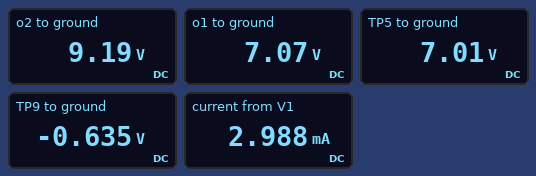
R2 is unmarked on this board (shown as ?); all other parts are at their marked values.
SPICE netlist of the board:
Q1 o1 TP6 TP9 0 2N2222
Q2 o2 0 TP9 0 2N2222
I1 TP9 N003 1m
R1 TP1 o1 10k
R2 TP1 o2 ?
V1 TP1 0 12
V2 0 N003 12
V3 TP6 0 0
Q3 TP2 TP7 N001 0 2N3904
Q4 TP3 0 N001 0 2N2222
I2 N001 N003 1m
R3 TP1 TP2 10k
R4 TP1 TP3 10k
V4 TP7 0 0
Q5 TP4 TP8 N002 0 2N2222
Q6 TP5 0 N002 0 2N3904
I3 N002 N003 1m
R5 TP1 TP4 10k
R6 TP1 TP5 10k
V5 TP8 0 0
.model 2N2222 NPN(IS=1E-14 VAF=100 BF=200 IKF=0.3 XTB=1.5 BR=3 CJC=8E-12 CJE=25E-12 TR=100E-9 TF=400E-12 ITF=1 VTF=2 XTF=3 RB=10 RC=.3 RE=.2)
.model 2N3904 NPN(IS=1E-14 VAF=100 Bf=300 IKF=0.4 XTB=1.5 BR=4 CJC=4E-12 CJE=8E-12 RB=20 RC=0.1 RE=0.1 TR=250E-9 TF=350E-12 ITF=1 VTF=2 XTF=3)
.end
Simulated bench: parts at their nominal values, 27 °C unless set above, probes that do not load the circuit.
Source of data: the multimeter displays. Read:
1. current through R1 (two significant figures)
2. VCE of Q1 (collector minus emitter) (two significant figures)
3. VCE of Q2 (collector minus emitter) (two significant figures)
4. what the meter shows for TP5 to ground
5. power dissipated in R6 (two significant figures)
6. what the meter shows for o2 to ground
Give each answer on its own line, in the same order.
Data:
490 µA
7.7 V
9.8 V
7.01 V
2.5 mW
9.19 V
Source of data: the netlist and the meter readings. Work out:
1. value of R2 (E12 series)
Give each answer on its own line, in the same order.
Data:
5.6 kΩ
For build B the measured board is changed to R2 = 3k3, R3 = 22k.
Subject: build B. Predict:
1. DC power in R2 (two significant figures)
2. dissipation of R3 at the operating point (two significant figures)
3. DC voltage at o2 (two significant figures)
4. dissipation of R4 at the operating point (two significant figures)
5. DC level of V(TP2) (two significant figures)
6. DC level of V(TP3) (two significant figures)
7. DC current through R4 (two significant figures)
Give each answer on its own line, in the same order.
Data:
840 µW
5.2 mW
10 V
2.6 mW
1.3 V
6.9 V
510 µA
